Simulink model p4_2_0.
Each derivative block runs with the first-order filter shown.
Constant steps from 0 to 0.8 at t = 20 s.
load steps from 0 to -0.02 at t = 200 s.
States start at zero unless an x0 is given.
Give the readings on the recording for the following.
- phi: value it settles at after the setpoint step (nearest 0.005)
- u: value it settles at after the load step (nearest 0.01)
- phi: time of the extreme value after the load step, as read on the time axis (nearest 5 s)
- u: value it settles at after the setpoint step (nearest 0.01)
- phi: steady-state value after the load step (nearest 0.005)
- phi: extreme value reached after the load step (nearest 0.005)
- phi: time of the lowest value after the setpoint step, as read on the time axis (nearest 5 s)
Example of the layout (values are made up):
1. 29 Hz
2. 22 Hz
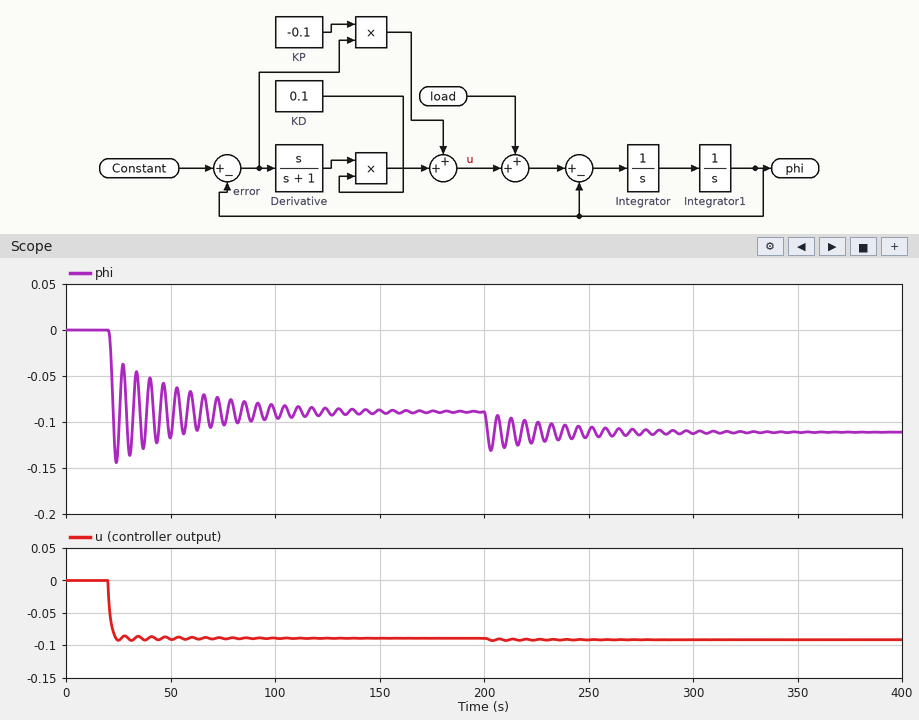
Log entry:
1. -0.090
2. -0.09
3. 205 s
4. -0.09
5. -0.110
6. -0.130
7. 25 s
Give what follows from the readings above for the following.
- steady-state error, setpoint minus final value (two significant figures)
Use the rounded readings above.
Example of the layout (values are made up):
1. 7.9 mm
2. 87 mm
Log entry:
1. 0.89
